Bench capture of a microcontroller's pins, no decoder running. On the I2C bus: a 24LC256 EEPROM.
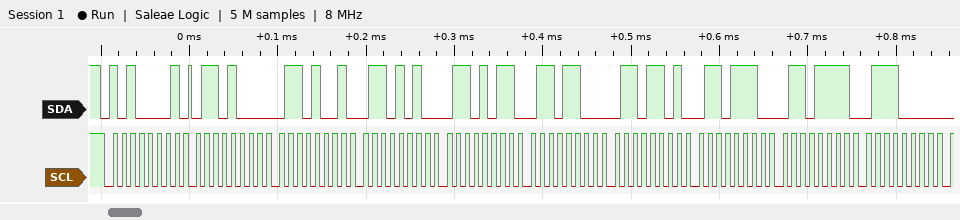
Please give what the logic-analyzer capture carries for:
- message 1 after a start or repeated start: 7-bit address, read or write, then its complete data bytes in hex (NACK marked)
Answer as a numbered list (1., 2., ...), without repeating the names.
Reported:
1. 0x50 read: 68 69 6A 6B 6C 6D 6E 6F 70
